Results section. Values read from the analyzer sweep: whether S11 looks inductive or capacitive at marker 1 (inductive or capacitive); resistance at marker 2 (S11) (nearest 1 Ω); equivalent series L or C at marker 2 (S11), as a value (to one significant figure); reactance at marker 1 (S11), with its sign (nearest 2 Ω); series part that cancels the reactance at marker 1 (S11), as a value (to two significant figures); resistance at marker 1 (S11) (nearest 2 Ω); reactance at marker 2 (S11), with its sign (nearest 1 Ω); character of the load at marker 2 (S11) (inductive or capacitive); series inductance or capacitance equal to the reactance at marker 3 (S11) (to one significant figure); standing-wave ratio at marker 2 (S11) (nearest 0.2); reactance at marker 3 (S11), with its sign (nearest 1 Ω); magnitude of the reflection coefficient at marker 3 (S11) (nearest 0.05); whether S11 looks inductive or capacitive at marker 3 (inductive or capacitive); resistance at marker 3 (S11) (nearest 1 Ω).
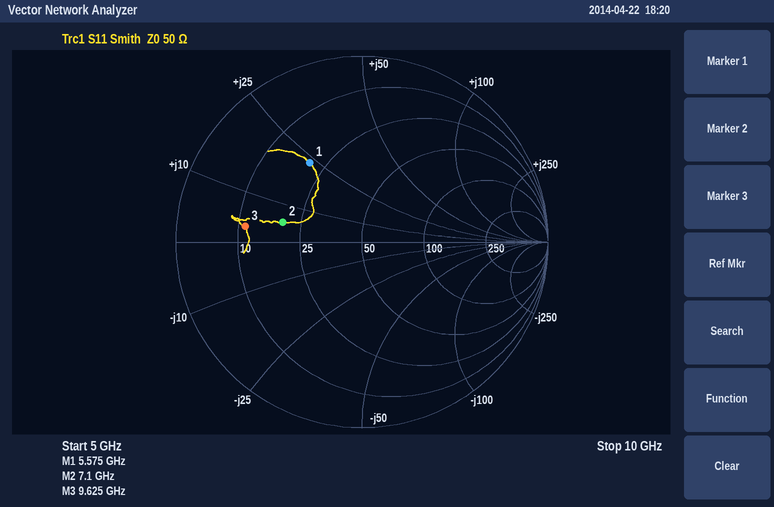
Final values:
inductive
20 Ω
100 pH
+24 Ω
1.2 pF
20 Ω
+5 Ω
inductive
50 pH
2.6
+3 Ω
0.65
inductive
11 Ω
